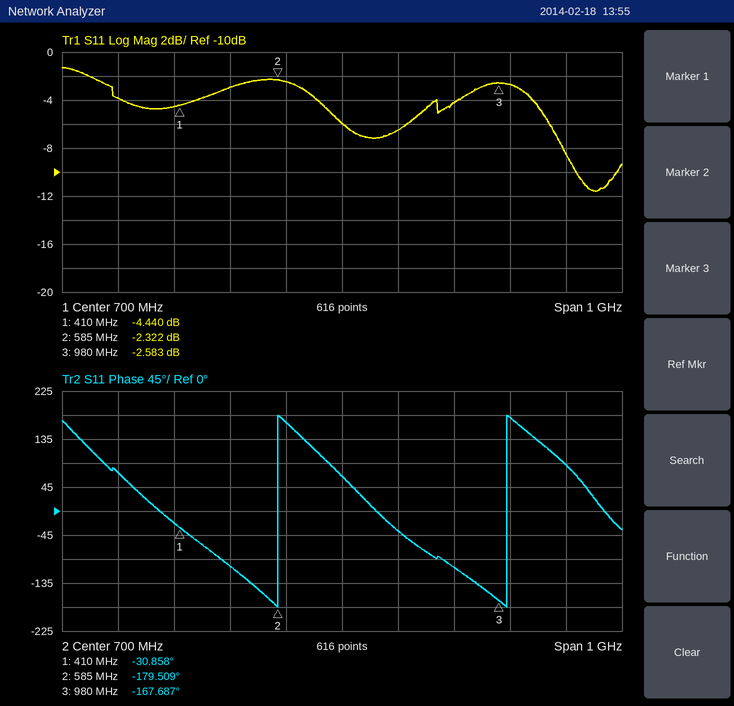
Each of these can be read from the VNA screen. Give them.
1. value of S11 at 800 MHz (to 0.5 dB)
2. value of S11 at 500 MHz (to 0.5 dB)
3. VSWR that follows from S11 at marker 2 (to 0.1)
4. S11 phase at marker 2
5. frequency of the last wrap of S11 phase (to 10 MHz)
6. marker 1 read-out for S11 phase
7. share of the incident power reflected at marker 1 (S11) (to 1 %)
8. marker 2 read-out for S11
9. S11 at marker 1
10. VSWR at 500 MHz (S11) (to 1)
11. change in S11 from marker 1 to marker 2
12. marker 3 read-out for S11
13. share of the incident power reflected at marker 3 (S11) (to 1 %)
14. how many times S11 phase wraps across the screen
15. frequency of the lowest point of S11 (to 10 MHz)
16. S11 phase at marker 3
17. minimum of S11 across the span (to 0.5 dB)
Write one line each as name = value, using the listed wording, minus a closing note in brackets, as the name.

value of S11 at 800 MHz = -6.5 dB
value of S11 at 500 MHz = -3.0 dB
VSWR that follows from S11 at marker 2 = 7.5
S11 phase at marker 2 = -179.509°
frequency of the last wrap of S11 phase = 990 MHz
marker 1 read-out for S11 phase = -30.858°
share of the incident power reflected at marker 1 (S11) = 36 %
marker 2 read-out for S11 = -2.322 dB
S11 at marker 1 = -4.440 dB
VSWR at 500 MHz (S11) = 6
change in S11 from marker 1 to marker 2 = 2.118 dB
marker 3 read-out for S11 = -2.583 dB
share of the incident power reflected at marker 3 (S11) = 55 %
how many times S11 phase wraps across the screen = 2
frequency of the lowest point of S11 = 1.15 GHz
S11 phase at marker 3 = -167.687°
minimum of S11 across the span = -11.5 dB
